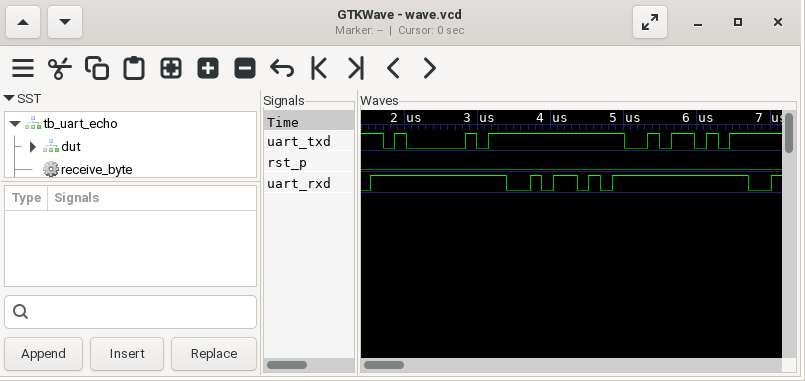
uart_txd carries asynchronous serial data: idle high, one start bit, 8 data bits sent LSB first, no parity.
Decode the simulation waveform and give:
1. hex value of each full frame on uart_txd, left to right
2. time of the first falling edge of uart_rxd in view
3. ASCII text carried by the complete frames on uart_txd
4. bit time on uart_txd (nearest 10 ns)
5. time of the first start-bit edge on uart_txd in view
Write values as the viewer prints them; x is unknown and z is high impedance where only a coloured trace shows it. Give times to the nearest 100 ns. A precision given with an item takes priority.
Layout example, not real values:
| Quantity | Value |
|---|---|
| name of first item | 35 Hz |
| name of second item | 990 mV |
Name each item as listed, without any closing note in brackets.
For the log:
| Quantity | Value |
|---|---|
| hex value of each full frame on uart_txd, left to right | 41, 5A |
| time of the first falling edge of uart_rxd in view | 3400 ns |
| ASCII text carried by the complete frames on uart_txd | "AZ" |
| bit time on uart_txd | 160 ns |
| time of the first start-bit edge on uart_txd in view | 1700 ns |
